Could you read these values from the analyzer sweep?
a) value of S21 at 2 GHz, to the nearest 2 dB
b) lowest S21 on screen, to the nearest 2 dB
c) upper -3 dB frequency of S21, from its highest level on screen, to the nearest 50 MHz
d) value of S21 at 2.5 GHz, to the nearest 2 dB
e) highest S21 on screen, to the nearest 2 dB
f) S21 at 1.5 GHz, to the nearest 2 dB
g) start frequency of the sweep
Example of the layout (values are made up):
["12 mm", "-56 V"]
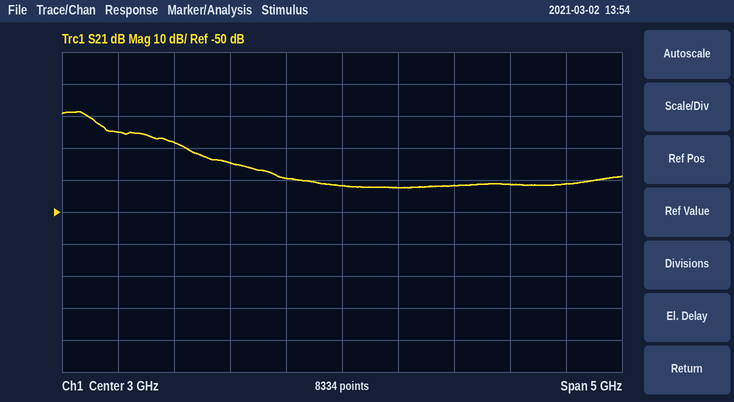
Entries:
["-34 dB", "-42 dB", "800 MHz", "-40 dB", "-18 dB", "-28 dB", "500 MHz"]
